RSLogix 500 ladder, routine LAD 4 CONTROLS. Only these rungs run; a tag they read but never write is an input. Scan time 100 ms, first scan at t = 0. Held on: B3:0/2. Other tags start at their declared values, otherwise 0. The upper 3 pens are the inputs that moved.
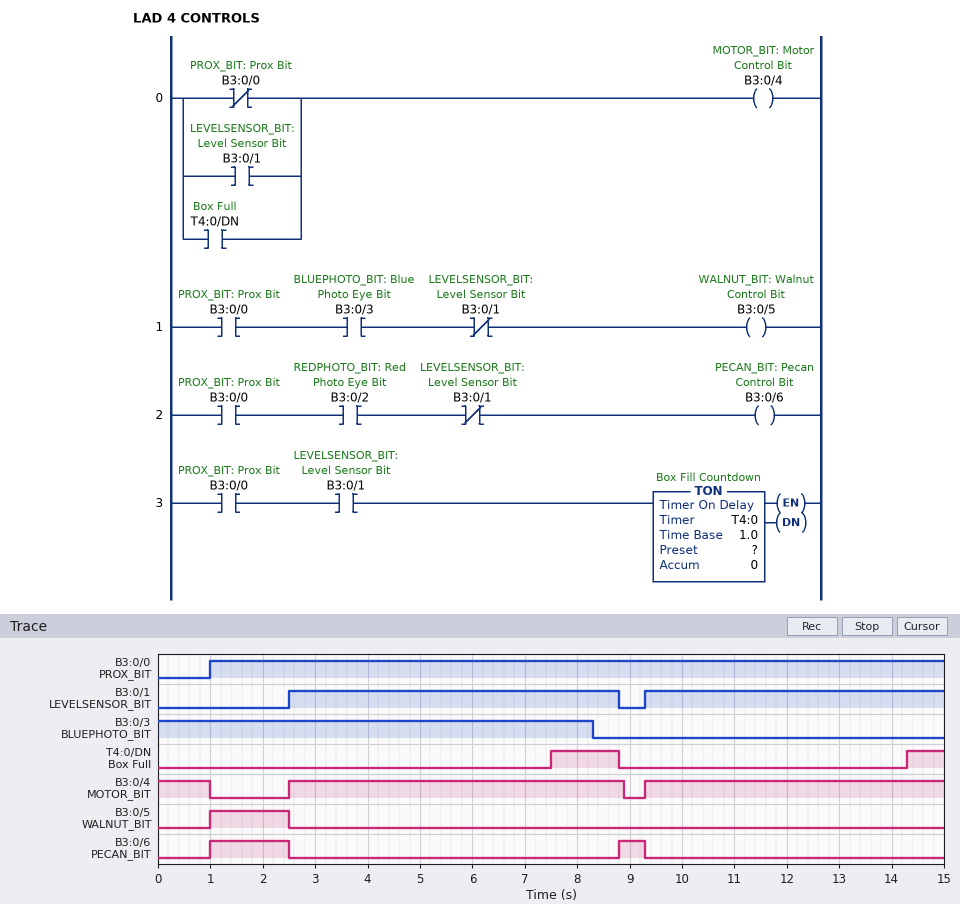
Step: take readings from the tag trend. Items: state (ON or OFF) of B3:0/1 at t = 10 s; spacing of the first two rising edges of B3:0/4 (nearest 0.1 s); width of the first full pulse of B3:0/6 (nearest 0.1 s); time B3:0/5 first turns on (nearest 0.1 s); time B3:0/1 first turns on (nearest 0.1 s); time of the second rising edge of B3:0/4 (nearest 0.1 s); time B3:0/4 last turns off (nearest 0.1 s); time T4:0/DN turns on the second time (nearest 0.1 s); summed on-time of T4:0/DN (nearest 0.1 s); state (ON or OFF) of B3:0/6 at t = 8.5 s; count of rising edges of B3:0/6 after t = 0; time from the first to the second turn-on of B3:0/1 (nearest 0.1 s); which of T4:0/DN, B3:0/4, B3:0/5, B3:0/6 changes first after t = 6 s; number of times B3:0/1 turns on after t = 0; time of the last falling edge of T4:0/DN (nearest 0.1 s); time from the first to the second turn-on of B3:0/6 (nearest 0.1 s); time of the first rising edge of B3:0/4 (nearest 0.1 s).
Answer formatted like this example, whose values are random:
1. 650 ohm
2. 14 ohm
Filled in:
1. ON
2. 6.8 s
3. 1.5 s
4. 1.0 s
5. 2.5 s
6. 9.3 s
7. 8.9 s
8. 14.3 s
9. 2.0 s
10. OFF
11. 2
12. 6.8 s
13. T4:0/DN
14. 2
15. 8.8 s
16. 7.8 s
17. 2.5 s
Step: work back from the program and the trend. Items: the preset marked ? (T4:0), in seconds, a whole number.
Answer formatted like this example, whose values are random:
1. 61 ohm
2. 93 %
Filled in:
1. 5 s
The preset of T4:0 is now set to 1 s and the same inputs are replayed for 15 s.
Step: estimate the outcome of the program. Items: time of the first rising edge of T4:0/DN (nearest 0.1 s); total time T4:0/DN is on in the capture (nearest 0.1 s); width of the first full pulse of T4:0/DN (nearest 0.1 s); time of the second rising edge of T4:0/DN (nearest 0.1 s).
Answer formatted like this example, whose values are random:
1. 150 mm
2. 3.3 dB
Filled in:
1. 3.5 s
2. 10.0 s
3. 5.3 s
4. 10.3 s
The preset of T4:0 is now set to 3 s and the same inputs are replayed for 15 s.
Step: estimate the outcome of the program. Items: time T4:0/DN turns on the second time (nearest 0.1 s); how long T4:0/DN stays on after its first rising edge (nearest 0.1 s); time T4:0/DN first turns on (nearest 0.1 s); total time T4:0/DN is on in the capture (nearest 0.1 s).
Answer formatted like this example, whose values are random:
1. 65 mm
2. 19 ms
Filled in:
1. 12.3 s
2. 3.3 s
3. 5.5 s
4. 6.0 s
